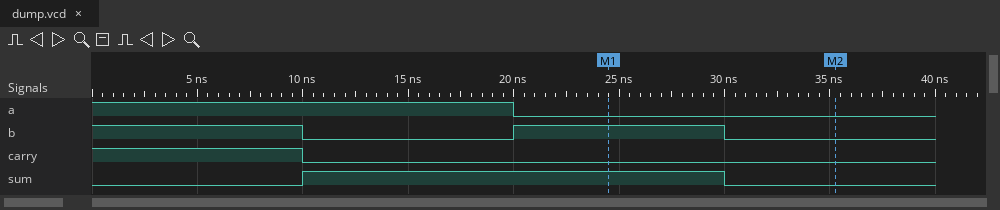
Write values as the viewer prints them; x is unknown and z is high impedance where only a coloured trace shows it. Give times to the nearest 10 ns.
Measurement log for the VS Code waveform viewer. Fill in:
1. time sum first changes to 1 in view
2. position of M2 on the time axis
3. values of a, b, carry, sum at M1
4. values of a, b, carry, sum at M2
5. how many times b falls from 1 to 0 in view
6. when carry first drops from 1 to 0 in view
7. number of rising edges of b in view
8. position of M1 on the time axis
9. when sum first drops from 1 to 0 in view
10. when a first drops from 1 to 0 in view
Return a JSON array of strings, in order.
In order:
["10 ns", "40 ns", "a=0, b=1, carry=0, sum=1", "a=0, b=0, carry=0, sum=0", "2", "10 ns", "1", "20 ns", "30 ns", "20 ns"]
